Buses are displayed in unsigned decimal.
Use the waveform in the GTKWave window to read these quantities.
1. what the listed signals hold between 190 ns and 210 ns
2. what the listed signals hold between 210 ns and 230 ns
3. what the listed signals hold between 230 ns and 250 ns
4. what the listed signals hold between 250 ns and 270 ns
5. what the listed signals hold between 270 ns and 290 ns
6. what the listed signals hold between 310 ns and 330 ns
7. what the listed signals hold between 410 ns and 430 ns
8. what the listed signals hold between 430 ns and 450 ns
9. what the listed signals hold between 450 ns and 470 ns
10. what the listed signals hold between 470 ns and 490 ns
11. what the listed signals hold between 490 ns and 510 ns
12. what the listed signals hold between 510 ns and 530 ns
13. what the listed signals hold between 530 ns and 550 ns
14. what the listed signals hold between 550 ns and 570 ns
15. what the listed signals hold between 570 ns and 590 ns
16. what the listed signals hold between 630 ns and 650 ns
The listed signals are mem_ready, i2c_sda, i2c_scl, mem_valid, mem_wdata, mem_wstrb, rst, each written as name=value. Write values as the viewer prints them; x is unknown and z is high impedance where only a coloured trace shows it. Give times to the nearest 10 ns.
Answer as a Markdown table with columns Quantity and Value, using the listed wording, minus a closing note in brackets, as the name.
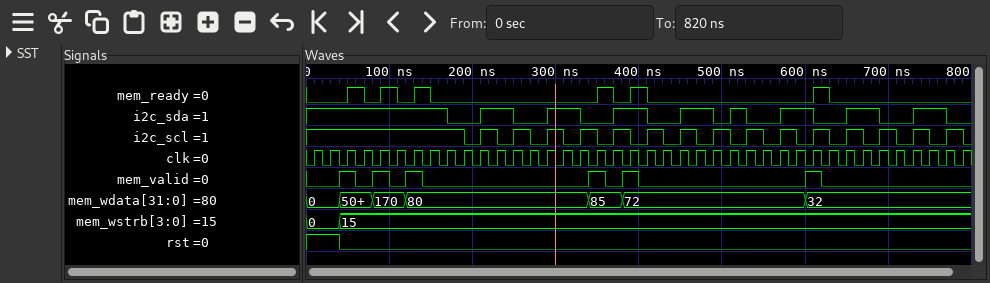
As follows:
| Quantity | Value |
|---|---|
| what the listed signals hold between 190 ns and 210 ns | mem_ready=0, i2c_sda=0, i2c_scl=0, mem_valid=0, mem_wdata=80, mem_wstrb=15, rst=0 |
| what the listed signals hold between 210 ns and 230 ns | mem_ready=0, i2c_sda=1, i2c_scl=1, mem_valid=0, mem_wdata=80, mem_wstrb=15, rst=0 |
| what the listed signals hold between 230 ns and 250 ns | mem_ready=0, i2c_sda=1, i2c_scl=0, mem_valid=0, mem_wdata=80, mem_wstrb=15, rst=0 |
| what the listed signals hold between 250 ns and 270 ns | mem_ready=0, i2c_sda=0, i2c_scl=1, mem_valid=0, mem_wdata=80, mem_wstrb=15, rst=0 |
| what the listed signals hold between 270 ns and 290 ns | mem_ready=0, i2c_sda=0, i2c_scl=0, mem_valid=0, mem_wdata=80, mem_wstrb=15, rst=0 |
| what the listed signals hold between 310 ns and 330 ns | mem_ready=0, i2c_sda=1, i2c_scl=0, mem_valid=0, mem_wdata=80, mem_wstrb=15, rst=0 |
| what the listed signals hold between 410 ns and 430 ns | mem_ready=0, i2c_sda=0, i2c_scl=1, mem_valid=0, mem_wdata=72, mem_wstrb=15, rst=0 |
| what the listed signals hold between 430 ns and 450 ns | mem_ready=0, i2c_sda=0, i2c_scl=0, mem_valid=0, mem_wdata=72, mem_wstrb=15, rst=0 |
| what the listed signals hold between 450 ns and 470 ns | mem_ready=0, i2c_sda=1, i2c_scl=1, mem_valid=0, mem_wdata=72, mem_wstrb=15, rst=0 |
| what the listed signals hold between 470 ns and 490 ns | mem_ready=0, i2c_sda=1, i2c_scl=0, mem_valid=0, mem_wdata=72, mem_wstrb=15, rst=0 |
| what the listed signals hold between 490 ns and 510 ns | mem_ready=0, i2c_sda=0, i2c_scl=1, mem_valid=0, mem_wdata=72, mem_wstrb=15, rst=0 |
| what the listed signals hold between 510 ns and 530 ns | mem_ready=0, i2c_sda=1, i2c_scl=0, mem_valid=0, mem_wdata=72, mem_wstrb=15, rst=0 |
| what the listed signals hold between 530 ns and 550 ns | mem_ready=0, i2c_sda=0, i2c_scl=1, mem_valid=0, mem_wdata=72, mem_wstrb=15, rst=0 |
| what the listed signals hold between 550 ns and 570 ns | mem_ready=0, i2c_sda=0, i2c_scl=0, mem_valid=0, mem_wdata=72, mem_wstrb=15, rst=0 |
| what the listed signals hold between 570 ns and 590 ns | mem_ready=0, i2c_sda=1, i2c_scl=1, mem_valid=0, mem_wdata=72, mem_wstrb=15, rst=0 |
| what the listed signals hold between 630 ns and 650 ns | mem_ready=0, i2c_sda=0, i2c_scl=0, mem_valid=0, mem_wdata=32, mem_wstrb=15, rst=0 |
